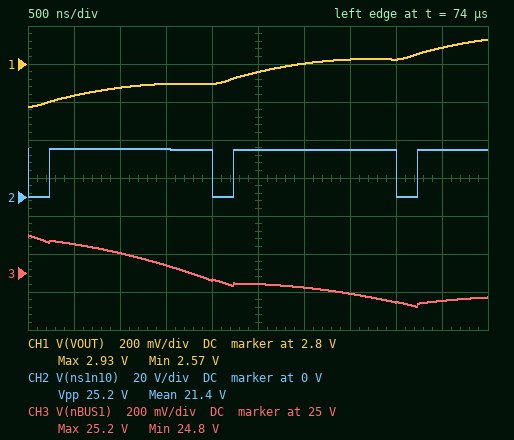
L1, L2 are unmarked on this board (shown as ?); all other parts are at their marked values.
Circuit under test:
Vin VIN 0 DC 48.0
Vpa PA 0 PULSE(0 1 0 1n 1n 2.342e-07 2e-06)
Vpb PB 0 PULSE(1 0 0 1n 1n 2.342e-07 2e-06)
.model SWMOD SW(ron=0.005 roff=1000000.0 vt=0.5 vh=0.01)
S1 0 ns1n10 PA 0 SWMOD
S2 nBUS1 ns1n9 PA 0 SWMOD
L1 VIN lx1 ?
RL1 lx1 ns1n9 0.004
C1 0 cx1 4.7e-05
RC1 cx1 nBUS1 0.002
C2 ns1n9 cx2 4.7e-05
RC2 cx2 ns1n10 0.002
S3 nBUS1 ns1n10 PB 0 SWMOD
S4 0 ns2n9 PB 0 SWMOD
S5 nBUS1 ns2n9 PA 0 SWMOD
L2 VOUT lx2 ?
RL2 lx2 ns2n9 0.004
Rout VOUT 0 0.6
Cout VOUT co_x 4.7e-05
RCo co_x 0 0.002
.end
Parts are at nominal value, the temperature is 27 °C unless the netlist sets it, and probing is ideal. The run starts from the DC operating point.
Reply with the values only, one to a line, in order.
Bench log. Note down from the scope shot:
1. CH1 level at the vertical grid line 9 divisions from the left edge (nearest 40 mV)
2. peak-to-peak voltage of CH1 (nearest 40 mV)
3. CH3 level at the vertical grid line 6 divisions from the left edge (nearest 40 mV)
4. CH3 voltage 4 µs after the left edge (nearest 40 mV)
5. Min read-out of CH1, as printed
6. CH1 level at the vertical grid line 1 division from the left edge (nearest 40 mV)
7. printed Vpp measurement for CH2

2.88 V
360 mV
24.92 V
24.84 V
2.57 V
2.64 V
25.2 V
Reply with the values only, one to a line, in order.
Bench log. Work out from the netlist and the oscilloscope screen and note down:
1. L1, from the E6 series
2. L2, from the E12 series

680 nH
680 nH
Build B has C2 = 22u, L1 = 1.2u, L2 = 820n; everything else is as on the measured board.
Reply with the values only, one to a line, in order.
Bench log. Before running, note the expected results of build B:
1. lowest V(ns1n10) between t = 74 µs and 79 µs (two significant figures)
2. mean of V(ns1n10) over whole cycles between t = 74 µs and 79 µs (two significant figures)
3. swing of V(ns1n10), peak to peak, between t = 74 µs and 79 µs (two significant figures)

-170 mV
24 V
27 V
